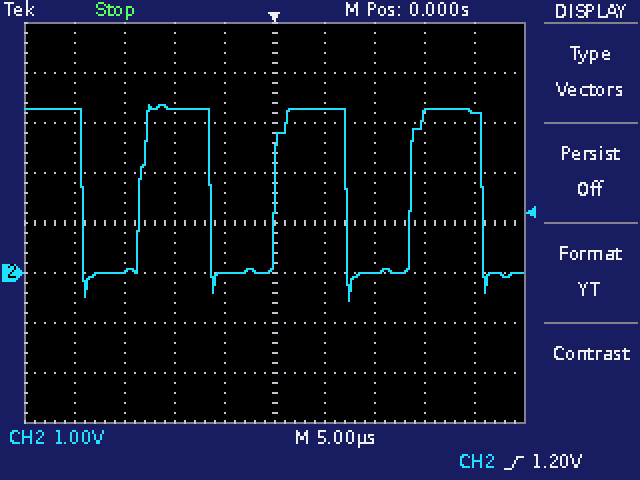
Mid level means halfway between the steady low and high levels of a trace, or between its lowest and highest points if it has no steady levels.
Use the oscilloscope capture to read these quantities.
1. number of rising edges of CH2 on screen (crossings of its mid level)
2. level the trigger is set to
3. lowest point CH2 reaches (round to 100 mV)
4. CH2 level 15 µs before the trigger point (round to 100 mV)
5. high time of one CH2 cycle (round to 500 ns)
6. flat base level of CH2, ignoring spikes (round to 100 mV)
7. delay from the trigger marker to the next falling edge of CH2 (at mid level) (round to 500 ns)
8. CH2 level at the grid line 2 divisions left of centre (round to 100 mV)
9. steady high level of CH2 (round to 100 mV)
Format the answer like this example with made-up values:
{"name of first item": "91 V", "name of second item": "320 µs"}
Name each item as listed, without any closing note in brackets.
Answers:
{"number of rising edges of CH2 on screen": "3", "level the trigger is set to": "1.20 V", "lowest point CH2 reaches": "-600 mV", "CH2 level 15 µs before the trigger point": "0.0 V", "high time of one CH2 cycle": "7.0 µs", "flat base level of CH2, ignoring spikes": "0.0 V", "delay from the trigger marker to the next falling edge of CH2 (at mid level)": "7.0 µs", "CH2 level at the grid line 2 divisions left of centre": "3.3 V", "steady high level of CH2": "3.3 V"}
